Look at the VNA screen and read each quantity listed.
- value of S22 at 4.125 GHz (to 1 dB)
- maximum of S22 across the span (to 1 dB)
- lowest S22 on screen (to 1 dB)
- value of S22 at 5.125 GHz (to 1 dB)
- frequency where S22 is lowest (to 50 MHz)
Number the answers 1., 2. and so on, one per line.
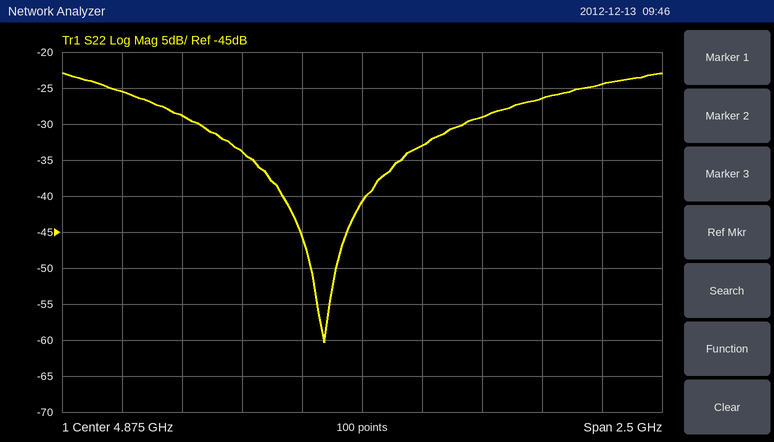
1. -29 dB
2. -23 dB
3. -60 dB
4. -33 dB
5. 4.70 GHz
